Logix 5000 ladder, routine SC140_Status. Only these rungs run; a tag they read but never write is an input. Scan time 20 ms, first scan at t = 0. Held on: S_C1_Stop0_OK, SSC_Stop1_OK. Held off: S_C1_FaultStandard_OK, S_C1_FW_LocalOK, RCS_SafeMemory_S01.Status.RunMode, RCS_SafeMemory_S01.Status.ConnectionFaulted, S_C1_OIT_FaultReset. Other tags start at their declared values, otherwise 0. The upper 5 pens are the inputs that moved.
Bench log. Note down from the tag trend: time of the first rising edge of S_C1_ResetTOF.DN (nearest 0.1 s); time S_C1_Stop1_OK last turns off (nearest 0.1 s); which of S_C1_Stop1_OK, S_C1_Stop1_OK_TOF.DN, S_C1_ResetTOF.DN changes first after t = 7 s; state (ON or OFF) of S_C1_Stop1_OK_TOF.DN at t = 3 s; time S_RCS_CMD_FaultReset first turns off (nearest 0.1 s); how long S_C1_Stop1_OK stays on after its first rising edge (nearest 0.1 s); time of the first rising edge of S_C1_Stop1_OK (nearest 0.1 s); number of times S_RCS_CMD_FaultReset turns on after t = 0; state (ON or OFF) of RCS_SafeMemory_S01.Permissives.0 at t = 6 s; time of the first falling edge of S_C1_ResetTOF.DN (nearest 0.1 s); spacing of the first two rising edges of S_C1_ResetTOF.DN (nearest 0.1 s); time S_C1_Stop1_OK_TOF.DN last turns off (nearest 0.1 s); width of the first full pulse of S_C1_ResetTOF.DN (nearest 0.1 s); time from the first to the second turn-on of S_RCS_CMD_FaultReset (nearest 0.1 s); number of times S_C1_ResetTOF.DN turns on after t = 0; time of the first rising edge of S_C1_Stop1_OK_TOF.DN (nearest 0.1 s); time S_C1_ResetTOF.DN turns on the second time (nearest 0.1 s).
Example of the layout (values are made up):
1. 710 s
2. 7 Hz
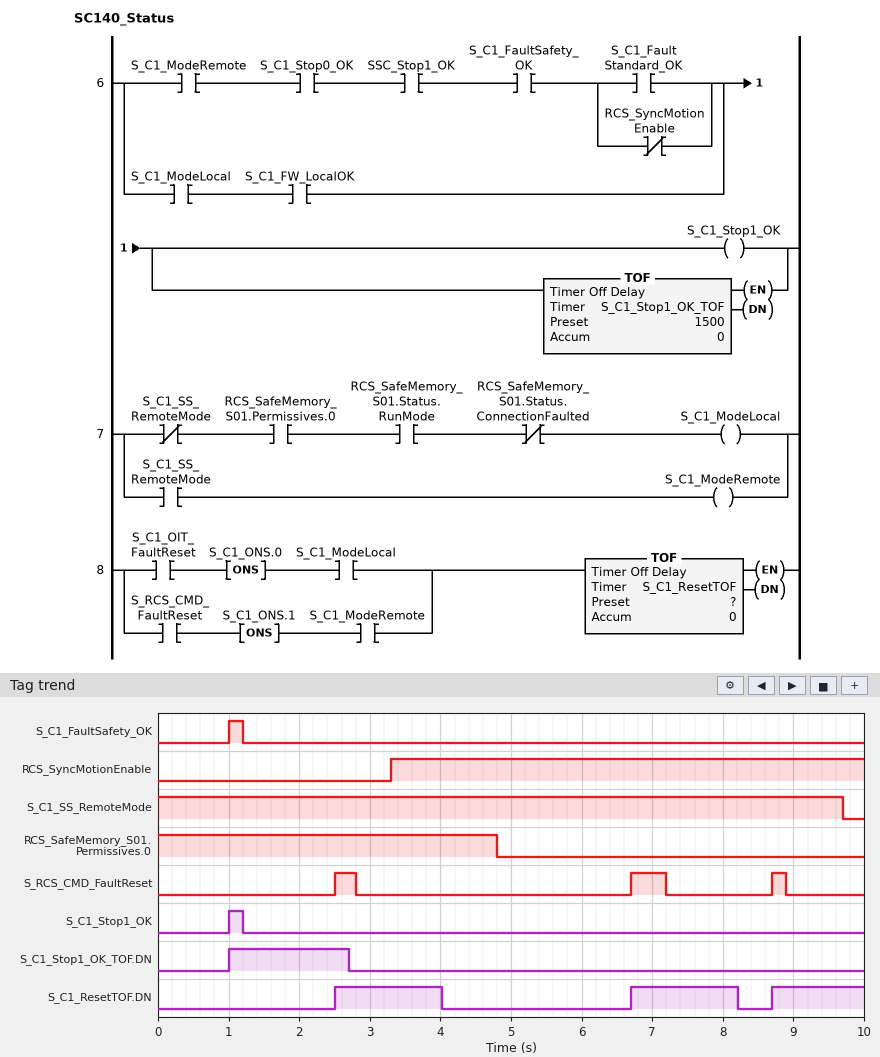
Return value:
1. 2.5 s
2. 1.2 s
3. S_C1_ResetTOF.DN
4. OFF
5. 2.8 s
6. 0.2 s
7. 1.0 s
8. 3
9. OFF
10. 4.0 s
11. 4.2 s
12. 2.7 s
13. 1.5 s
14. 4.2 s
15. 3
16. 1.0 s
17. 6.7 s
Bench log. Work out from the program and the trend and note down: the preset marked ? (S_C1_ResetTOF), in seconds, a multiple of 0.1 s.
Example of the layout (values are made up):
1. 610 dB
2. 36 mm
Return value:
1. 1.5 s
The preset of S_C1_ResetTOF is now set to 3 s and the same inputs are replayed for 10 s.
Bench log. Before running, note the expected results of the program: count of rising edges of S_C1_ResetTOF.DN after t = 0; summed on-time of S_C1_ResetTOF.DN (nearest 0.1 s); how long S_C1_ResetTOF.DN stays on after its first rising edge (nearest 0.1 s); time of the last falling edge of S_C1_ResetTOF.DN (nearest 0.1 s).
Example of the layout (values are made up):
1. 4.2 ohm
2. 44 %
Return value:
1. 2
2. 6.3 s
3. 3.0 s
4. 5.5 s
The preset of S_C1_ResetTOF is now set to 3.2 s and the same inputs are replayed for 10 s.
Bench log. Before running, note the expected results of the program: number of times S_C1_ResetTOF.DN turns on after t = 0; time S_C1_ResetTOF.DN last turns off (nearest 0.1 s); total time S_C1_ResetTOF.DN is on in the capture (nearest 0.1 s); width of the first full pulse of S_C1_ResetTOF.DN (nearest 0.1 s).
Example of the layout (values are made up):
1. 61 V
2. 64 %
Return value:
1. 2
2. 5.7 s
3. 6.5 s
4. 3.2 s
